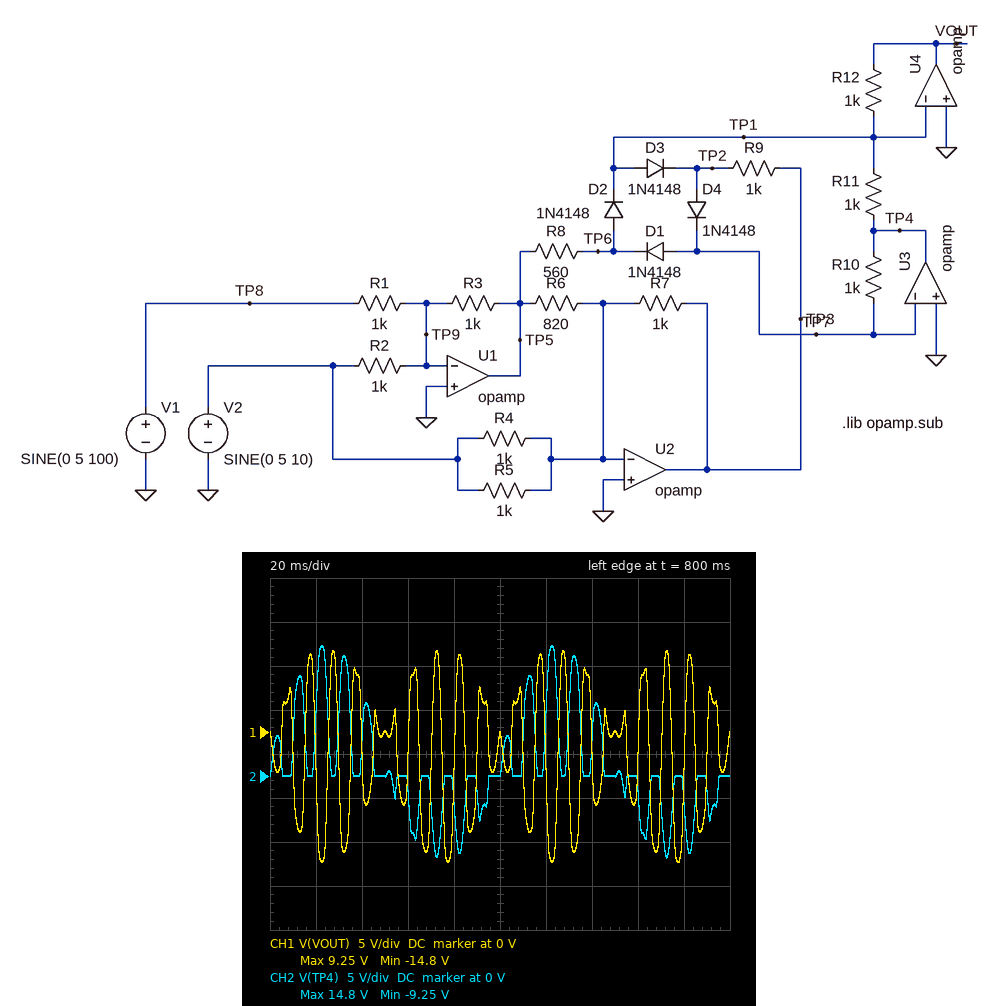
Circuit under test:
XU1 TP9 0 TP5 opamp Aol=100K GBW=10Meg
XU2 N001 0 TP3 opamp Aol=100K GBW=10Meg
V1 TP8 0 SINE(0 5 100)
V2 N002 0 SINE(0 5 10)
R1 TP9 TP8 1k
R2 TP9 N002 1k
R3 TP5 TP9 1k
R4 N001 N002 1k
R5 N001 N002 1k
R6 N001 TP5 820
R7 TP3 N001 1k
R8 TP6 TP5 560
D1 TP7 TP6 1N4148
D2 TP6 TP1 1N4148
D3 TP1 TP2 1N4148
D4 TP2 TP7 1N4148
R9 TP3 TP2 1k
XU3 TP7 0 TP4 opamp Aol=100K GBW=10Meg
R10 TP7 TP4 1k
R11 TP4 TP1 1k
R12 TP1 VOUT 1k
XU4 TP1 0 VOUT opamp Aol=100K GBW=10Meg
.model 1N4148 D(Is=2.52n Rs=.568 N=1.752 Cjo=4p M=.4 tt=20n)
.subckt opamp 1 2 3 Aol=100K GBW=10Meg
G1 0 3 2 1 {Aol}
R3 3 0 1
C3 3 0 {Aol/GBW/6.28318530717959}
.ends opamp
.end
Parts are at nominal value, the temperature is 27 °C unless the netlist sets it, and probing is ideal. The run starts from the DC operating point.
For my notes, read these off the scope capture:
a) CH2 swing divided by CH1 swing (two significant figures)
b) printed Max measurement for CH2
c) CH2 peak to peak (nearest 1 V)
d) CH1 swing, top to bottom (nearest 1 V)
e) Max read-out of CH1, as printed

1.0
14.8 V
24 V
24 V
9.25 V
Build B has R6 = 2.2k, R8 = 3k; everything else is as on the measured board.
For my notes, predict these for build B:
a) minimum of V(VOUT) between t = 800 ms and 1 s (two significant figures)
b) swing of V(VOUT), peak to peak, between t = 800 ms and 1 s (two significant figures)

-1.6 V
11 V
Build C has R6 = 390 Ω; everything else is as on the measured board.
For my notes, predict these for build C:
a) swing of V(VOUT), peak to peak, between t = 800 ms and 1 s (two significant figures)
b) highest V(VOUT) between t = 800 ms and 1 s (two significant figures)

16 V
9.5 V
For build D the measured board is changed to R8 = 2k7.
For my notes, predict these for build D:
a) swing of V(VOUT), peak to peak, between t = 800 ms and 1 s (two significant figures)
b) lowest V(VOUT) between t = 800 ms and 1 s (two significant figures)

12 V
-2.9 V
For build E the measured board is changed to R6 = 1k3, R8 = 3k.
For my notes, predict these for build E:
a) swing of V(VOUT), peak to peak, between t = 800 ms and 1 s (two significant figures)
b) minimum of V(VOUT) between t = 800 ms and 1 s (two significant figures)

12 V
-2.6 V
